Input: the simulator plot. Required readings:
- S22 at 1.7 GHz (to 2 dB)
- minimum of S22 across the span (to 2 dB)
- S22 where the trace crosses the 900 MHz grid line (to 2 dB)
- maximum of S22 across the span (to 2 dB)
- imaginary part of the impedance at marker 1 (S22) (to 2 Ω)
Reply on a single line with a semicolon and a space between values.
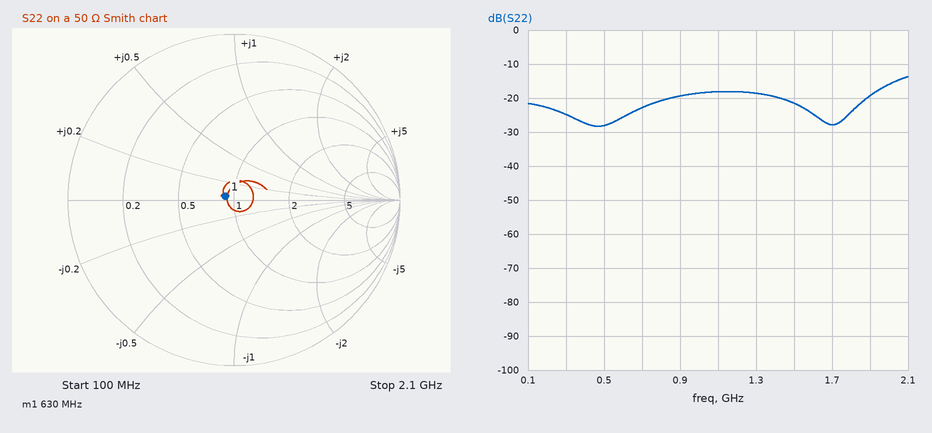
-28 dB; -28 dB; -20 dB; -14 dB; +2 Ω
